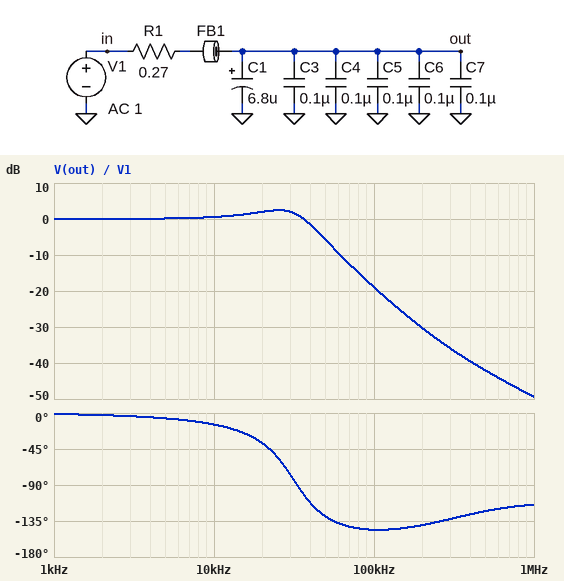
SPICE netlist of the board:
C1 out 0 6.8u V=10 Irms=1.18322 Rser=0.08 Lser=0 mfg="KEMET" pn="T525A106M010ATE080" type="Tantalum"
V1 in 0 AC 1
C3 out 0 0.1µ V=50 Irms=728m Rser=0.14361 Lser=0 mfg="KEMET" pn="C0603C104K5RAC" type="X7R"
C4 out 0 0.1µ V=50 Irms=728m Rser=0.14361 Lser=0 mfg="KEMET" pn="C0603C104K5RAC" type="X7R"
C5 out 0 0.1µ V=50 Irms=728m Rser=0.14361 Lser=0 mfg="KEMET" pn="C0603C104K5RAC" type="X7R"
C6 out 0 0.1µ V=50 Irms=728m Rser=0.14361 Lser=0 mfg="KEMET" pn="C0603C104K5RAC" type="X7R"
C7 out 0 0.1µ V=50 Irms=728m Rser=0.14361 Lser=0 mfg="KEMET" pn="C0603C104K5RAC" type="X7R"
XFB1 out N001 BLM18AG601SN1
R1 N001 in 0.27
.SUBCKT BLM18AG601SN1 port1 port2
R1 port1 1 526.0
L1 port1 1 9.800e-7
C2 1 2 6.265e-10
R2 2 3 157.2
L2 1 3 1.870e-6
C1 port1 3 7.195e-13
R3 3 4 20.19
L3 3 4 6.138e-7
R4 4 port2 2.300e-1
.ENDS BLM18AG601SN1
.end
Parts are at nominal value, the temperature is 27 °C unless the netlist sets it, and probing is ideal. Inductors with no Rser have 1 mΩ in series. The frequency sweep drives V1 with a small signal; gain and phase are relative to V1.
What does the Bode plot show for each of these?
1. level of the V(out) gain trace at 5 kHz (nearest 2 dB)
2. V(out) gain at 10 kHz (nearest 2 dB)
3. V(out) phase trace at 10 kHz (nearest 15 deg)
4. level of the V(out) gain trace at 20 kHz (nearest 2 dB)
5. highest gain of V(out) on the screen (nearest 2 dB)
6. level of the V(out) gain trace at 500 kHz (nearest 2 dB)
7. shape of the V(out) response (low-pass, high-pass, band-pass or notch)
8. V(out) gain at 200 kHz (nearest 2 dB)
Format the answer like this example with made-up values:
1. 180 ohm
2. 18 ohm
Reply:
1. 0 dB
2. 0 dB
3. -15 deg
4. 2 dB
5. 2 dB
6. -42 dB
7. low-pass
8. -30 dB
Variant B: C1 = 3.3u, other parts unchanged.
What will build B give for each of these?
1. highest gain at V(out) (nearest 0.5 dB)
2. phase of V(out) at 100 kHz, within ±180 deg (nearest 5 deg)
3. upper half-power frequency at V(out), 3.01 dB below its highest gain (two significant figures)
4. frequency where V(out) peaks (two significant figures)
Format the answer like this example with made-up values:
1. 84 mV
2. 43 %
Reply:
1. 5.0 dB
2. -155 deg
3. 52 kHz
4. 40 kHz
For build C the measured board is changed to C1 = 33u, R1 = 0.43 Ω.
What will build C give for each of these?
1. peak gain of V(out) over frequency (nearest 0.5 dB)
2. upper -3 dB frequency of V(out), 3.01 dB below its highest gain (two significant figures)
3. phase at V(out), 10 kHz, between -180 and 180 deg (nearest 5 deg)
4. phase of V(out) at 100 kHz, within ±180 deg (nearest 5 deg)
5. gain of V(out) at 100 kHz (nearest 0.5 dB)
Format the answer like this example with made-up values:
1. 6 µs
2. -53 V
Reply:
1. 0 dB
2. 7.9 kHz
3. -60 deg
4. -105 deg
5. -28.0 dB
